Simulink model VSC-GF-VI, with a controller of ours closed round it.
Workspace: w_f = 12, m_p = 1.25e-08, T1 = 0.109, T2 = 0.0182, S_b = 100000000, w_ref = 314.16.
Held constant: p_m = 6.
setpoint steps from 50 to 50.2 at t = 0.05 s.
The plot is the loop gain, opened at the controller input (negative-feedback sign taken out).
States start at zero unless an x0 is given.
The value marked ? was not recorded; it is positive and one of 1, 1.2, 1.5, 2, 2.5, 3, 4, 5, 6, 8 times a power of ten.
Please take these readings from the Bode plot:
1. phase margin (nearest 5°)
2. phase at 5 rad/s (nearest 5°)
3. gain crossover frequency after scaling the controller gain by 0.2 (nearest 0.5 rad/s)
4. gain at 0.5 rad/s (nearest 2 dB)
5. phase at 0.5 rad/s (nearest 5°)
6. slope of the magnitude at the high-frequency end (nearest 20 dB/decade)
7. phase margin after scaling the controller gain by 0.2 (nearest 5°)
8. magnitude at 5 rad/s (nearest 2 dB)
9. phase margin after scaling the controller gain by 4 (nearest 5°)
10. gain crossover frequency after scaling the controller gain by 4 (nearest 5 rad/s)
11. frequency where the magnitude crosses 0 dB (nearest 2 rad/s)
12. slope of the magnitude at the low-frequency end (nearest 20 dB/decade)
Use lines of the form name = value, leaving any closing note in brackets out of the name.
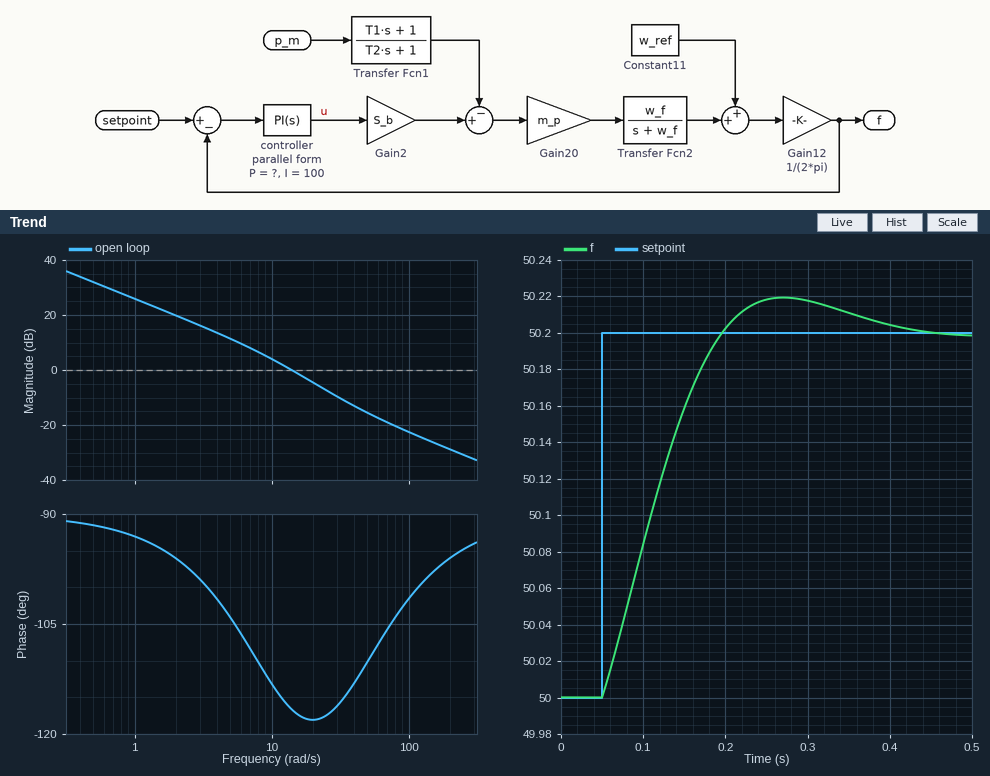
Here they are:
phase margin = 65°
phase at 5 rad/s = -105°
gain crossover frequency after scaling the controller gain by 0.2 = 4.0 rad/s
gain at 0.5 rad/s = 32 dB
phase at 0.5 rad/s = -90°
slope of the magnitude at the high-frequency end = -20 dB/decade
phase margin after scaling the controller gain by 0.2 = 80°
magnitude at 5 rad/s = 12 dB
phase margin after scaling the controller gain by 4 = 65°
gain crossover frequency after scaling the controller gain by 4 = 35 rad/s
frequency where the magnitude crosses 0 dB = 14 rad/s
slope of the magnitude at the low-frequency end = -20 dB/decade
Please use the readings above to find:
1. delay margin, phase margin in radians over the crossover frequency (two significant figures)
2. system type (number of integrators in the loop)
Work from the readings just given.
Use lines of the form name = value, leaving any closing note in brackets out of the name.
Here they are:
delay margin, phase margin in radians over the crossover frequency = 0.081 s
system type = 1
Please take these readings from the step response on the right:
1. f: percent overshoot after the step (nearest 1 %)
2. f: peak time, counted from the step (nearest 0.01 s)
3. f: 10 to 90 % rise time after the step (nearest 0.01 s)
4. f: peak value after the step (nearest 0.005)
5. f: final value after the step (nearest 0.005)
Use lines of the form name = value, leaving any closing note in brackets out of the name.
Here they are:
f: percent overshoot after the step = 10 %
f: peak time, counted from the step = 0.22 s
f: 10 to 90 % rise time after the step = 0.11 s
f: peak value after the step = 50.220
f: final value after the step = 50.200
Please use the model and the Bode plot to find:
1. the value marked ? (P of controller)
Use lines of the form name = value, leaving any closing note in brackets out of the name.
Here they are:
the value marked ? = 3
